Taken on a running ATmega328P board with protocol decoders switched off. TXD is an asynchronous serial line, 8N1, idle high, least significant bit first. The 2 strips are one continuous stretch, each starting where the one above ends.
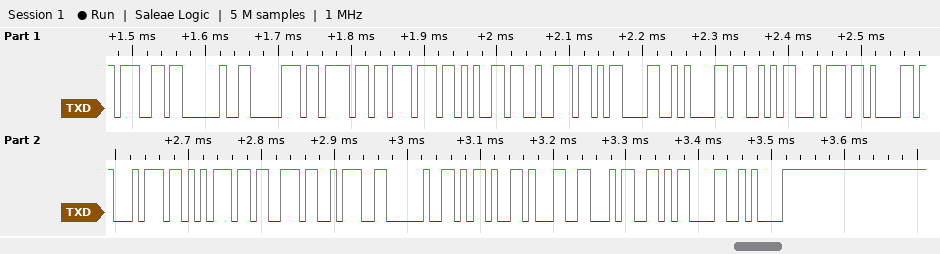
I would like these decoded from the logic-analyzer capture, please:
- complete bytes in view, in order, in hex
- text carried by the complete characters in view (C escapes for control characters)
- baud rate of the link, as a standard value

67 20 70 6F 77 65 72 0D 0A 53 74 61 74 75 73 3A 20 2D 31 34 0D 0A
"g power\r\nStatus: -14\r\n"
115200 baud
